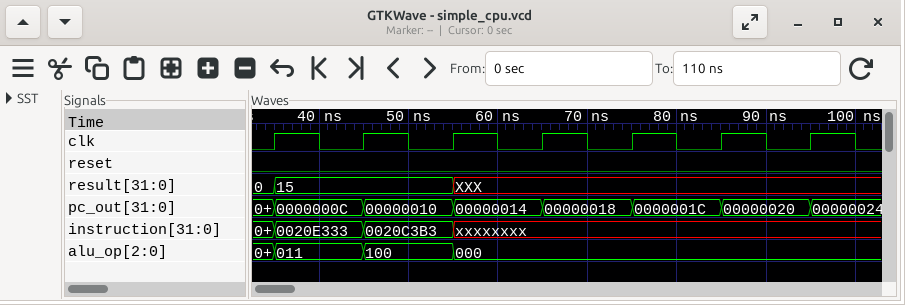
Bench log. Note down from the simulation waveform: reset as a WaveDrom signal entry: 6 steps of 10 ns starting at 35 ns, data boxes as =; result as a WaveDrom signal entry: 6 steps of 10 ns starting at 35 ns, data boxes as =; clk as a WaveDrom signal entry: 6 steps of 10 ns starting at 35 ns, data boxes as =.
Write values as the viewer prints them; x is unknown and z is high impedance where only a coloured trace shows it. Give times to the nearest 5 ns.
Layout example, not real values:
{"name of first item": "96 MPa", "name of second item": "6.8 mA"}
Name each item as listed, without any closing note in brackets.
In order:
{"reset as a WaveDrom signal entry: 6 steps of 10 ns starting at 35 ns, data boxes as =": "{name: 'reset', wave: '0.....'}", "result as a WaveDrom signal entry: 6 steps of 10 ns starting at 35 ns, data boxes as =": "{name: 'result', wave: '=.x...', data: '15'}", "clk as a WaveDrom signal entry: 6 steps of 10 ns starting at 35 ns, data boxes as =": "{name: 'clk', wave: 'p.....'}"}
